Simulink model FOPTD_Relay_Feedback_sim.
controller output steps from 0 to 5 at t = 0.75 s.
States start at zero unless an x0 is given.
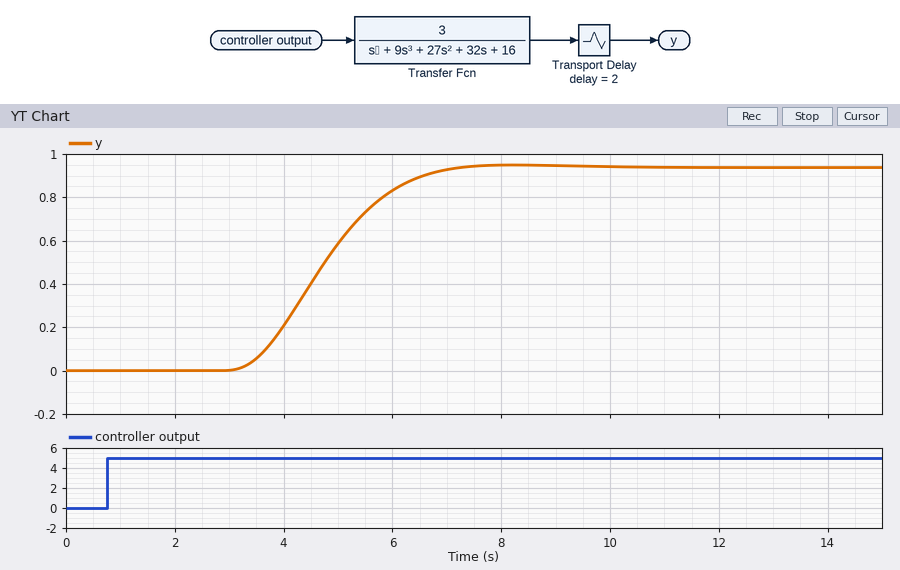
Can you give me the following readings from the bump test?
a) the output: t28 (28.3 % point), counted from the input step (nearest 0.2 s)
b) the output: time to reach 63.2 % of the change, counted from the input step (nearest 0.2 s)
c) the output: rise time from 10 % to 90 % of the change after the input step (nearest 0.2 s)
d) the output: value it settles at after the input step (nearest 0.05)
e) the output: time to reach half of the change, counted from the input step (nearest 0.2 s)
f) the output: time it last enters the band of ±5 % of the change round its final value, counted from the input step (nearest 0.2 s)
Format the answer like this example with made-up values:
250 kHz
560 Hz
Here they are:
3.4 s
4.2 s
2.4 s
0.95
4.0 s
5.8 s
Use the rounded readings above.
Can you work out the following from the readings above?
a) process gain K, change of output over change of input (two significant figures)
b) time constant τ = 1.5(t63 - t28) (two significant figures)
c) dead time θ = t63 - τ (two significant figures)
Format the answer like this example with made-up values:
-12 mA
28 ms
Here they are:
0.19
1.2 s
3.0 s
